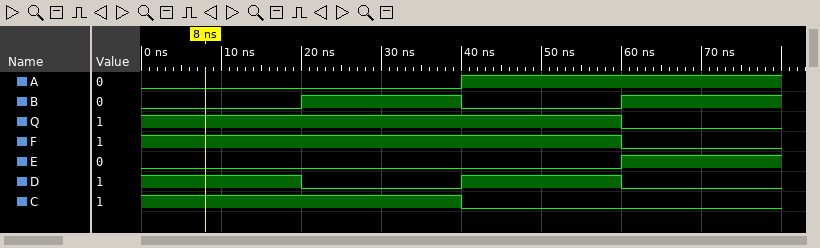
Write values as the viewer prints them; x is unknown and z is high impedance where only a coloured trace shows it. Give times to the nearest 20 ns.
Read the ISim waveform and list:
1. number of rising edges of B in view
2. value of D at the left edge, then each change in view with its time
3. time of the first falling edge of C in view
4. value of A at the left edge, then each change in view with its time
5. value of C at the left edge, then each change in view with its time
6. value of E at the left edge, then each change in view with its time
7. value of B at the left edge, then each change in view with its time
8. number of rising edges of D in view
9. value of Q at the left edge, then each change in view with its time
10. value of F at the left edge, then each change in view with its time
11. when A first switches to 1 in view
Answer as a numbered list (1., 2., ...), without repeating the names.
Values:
1. 2
2. 1, 0 at 20 ns, 1 at 40 ns, 0 at 60 ns
3. 40 ns
4. 0, 1 at 40 ns
5. 1, 0 at 40 ns
6. 0, 1 at 60 ns
7. 0, 1 at 20 ns, 0 at 40 ns, 1 at 60 ns
8. 1
9. 1, 0 at 60 ns
10. 1, 0 at 60 ns
11. 40 ns
